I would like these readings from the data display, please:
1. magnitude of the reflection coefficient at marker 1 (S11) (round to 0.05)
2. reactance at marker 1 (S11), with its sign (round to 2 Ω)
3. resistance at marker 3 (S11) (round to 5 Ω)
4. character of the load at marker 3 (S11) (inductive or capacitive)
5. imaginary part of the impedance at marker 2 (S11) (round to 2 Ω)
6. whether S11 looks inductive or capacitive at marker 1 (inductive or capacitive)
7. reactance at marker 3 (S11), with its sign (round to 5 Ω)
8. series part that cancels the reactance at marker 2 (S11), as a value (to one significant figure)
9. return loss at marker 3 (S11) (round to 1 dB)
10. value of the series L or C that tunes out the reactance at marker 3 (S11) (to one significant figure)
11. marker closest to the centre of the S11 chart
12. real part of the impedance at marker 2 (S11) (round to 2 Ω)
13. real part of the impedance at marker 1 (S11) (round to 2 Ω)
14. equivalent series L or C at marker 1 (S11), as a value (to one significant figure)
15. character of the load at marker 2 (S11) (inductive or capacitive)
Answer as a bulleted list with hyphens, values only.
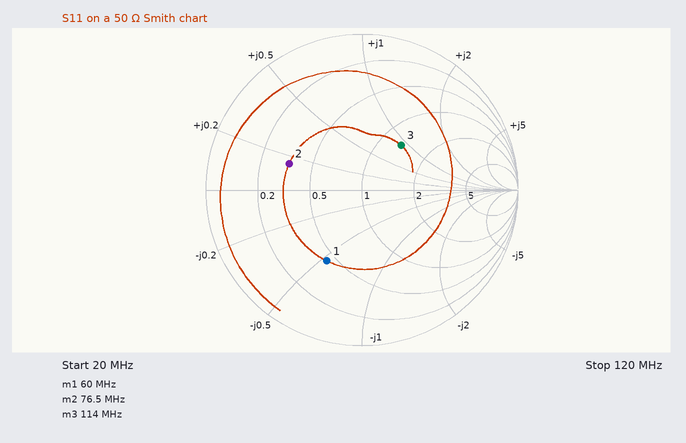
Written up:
- 0.50
- -26 Ω
- 65 Ω
- inductive
- +8 Ω
- capacitive
- +45 Ω
- 300 pF
- 8 dB
- 30 pF
- marker 3
- 18 Ω
- 22 Ω
- 100 pF
- inductive
